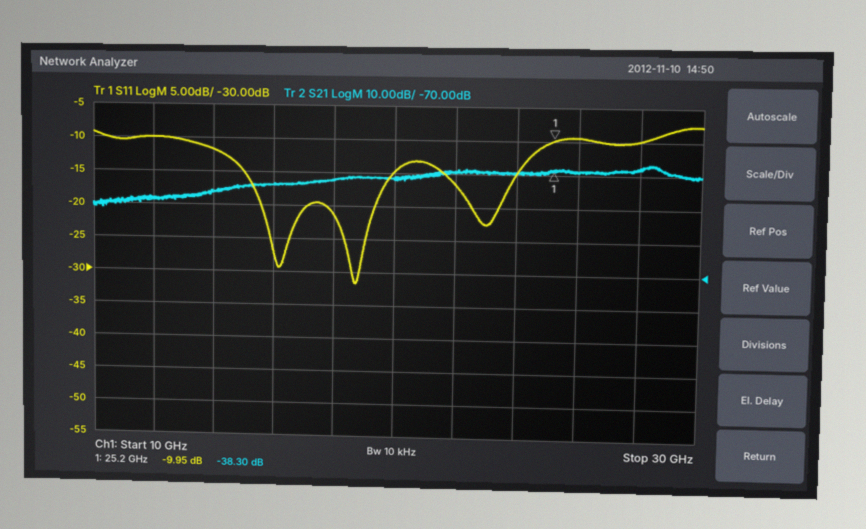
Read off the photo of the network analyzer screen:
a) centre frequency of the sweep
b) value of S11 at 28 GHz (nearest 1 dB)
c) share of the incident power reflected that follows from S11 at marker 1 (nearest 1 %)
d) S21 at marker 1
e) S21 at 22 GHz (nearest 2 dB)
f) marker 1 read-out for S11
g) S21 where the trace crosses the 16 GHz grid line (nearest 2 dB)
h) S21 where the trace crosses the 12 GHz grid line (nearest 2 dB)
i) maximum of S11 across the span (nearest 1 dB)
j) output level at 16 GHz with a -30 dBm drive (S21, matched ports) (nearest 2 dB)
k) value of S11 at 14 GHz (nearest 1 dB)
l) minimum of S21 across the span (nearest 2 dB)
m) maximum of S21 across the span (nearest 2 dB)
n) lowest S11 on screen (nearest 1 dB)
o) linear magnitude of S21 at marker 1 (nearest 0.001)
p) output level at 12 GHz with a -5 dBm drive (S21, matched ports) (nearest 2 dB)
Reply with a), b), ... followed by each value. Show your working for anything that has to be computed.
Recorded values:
a) 20 GHz
b) -10 dB
c) 10^(-9.95/10) ≈ 10 %
d) -38.30 dB
e) -40 dB
f) -9.95 dB
g) -44 dB
h) -48 dB
i) -8 dB
j) -30 dBm + (-44 dB) = -74 dBm
k) -12 dB
l) -52 dB
m) -36 dB
n) -32 dB
o) 10^(-38.3/20) ≈ 0.012
p) -5 dBm + (-48 dB) = -54 dBm
